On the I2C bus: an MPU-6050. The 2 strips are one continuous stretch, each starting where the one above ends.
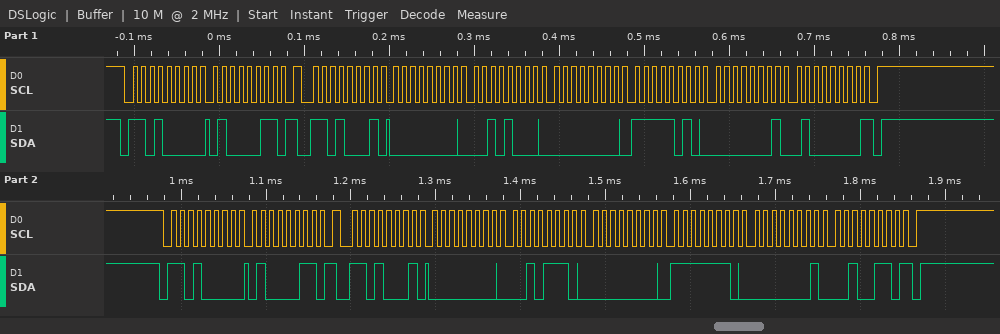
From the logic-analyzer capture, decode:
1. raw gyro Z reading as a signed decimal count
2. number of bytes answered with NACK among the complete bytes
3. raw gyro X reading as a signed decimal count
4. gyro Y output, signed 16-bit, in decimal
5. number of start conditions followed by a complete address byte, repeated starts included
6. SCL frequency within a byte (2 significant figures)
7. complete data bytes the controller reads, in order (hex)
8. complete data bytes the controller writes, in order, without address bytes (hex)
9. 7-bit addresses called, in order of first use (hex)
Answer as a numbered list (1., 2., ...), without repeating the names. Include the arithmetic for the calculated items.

1. 0x0140 = 320
2. 2
3. 0x0028 = 40
4. 0x00FA = 250
5. 4
6. 100 kHz
7. 00 28 00 FA 01 40 00 2E 00 FE 01 26
8. 43 43
9. 0x68
